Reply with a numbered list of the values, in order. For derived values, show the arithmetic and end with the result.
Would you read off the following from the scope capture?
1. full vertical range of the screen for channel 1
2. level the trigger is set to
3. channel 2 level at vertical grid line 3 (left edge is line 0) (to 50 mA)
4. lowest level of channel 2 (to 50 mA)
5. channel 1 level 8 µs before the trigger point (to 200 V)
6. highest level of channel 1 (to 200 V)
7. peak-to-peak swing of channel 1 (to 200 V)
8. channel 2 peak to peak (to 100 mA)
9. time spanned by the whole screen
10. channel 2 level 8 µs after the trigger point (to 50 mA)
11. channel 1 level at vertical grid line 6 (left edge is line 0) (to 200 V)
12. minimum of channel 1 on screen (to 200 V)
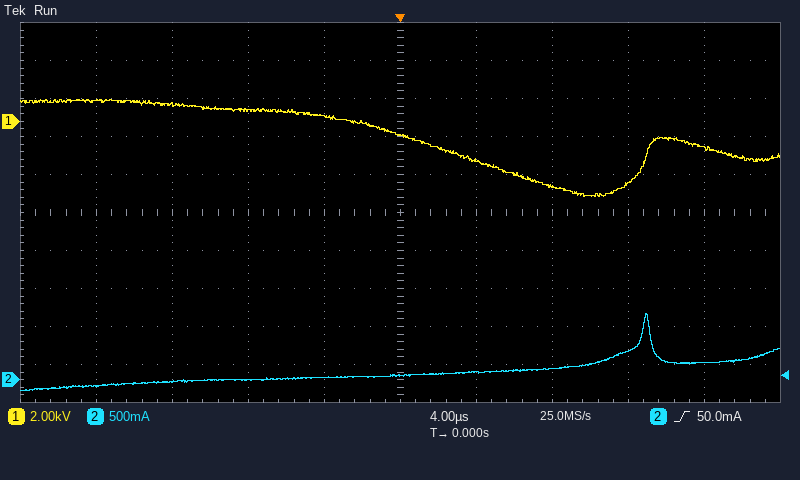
1. 20 kV
2. 50.0 mA
3. 0 mA
4. -150 mA
5. 600 V
6. 1.2 kV
7. 1.2 kV − (-4.0 kV) = 5.2 kV
8. 1.00 A
9. 40 µs
10. 150 mA
11. -2.0 kV
12. -4.0 kV
